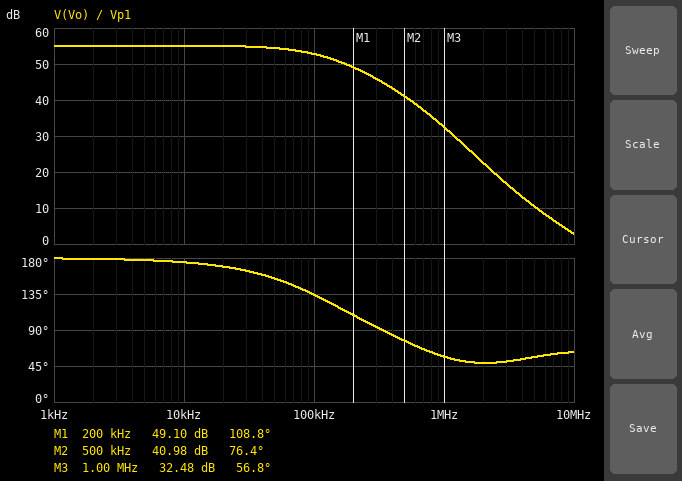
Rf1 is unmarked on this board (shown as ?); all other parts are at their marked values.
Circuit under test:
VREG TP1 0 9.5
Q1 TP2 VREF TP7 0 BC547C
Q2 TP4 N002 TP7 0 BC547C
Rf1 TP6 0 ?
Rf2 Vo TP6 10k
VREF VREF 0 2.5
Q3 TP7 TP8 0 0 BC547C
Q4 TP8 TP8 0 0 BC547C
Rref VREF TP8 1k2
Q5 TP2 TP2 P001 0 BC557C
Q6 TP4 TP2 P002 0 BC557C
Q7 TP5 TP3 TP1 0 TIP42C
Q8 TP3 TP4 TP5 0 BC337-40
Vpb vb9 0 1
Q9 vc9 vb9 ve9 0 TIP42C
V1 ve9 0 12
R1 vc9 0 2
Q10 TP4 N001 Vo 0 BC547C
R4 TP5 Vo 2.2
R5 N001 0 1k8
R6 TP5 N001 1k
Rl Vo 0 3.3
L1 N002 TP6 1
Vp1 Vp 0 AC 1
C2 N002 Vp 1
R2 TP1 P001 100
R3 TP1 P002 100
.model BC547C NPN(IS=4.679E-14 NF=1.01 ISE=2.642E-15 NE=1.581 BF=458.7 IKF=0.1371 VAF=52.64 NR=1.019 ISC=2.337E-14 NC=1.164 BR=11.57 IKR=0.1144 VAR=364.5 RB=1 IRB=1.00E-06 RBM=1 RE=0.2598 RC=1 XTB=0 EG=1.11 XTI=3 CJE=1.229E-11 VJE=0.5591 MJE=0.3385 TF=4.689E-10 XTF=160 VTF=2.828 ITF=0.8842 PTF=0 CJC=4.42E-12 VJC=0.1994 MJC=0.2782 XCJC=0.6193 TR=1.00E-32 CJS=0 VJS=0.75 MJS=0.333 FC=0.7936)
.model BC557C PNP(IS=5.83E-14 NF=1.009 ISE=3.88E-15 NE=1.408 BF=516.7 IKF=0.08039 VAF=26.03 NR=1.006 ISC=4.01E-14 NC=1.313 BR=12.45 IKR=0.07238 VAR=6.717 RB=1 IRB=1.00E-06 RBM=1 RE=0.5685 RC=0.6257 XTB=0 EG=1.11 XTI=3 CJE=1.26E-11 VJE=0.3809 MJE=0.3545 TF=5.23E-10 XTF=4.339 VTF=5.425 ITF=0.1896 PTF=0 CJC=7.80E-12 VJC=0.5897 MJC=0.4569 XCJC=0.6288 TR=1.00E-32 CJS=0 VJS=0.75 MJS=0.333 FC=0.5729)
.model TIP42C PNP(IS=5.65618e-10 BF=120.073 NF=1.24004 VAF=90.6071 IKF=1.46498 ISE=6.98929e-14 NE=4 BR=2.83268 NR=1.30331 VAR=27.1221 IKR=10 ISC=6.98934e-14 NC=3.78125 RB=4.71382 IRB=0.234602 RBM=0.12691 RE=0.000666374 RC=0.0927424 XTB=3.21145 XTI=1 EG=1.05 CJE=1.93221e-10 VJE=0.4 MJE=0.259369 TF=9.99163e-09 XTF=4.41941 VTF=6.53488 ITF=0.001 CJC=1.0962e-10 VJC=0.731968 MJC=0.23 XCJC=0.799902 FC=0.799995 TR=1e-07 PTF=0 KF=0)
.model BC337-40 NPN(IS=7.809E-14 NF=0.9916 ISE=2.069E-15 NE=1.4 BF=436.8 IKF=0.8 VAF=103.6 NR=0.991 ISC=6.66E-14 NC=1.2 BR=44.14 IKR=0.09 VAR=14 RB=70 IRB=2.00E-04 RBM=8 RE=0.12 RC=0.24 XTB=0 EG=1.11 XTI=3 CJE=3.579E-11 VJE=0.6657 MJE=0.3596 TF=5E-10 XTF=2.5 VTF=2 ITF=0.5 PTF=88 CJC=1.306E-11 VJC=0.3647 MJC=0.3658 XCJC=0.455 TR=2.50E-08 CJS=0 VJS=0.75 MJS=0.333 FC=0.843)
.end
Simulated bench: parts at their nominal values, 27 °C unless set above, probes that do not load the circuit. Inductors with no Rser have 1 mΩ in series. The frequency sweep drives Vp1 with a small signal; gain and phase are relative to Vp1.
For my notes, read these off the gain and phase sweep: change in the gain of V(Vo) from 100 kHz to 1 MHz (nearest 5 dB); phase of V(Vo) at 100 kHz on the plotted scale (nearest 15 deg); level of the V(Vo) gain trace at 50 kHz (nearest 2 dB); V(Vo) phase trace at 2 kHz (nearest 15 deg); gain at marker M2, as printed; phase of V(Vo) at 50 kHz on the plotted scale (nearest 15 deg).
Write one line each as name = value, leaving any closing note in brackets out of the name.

change in the gain of V(Vo) from 100 kHz to 1 MHz = -20 dB
phase of V(Vo) at 100 kHz on the plotted scale = 135 deg
level of the V(Vo) gain trace at 50 kHz = 54 dB
V(Vo) phase trace at 2 kHz = 180 deg
gain at marker M2, as printed = 40.98 dB
phase of V(Vo) at 50 kHz on the plotted scale = 150 deg
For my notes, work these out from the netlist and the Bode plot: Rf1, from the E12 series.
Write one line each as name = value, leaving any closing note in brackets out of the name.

Rf1, from the E12 series = 27 kΩ
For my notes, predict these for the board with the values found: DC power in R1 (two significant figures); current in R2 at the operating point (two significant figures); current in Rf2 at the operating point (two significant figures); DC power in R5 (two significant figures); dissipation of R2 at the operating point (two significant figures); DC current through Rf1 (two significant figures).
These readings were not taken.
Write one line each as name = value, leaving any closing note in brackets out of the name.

DC power in R1 = 65 W
current in R2 at the operating point = 800 µA
current in Rf2 at the operating point = 94 µA
DC power in R5 = 7.6 mW
dissipation of R2 at the operating point = 64 µW
DC current through Rf1 = 93 µA
